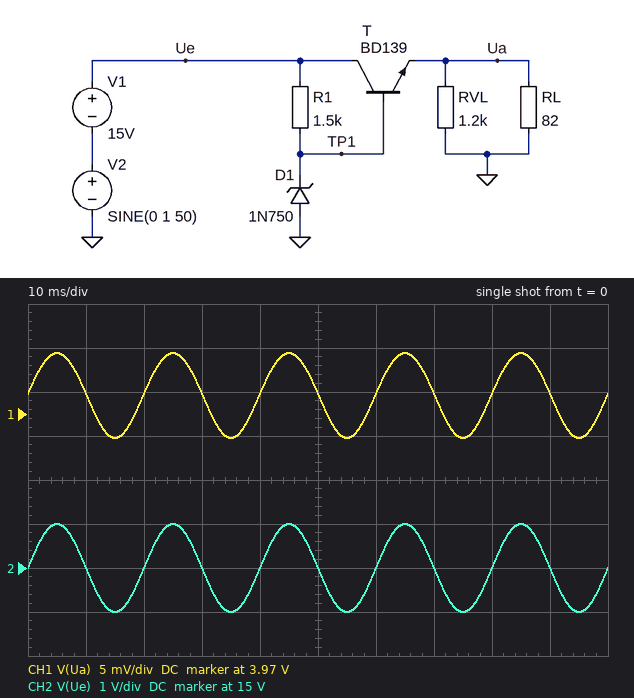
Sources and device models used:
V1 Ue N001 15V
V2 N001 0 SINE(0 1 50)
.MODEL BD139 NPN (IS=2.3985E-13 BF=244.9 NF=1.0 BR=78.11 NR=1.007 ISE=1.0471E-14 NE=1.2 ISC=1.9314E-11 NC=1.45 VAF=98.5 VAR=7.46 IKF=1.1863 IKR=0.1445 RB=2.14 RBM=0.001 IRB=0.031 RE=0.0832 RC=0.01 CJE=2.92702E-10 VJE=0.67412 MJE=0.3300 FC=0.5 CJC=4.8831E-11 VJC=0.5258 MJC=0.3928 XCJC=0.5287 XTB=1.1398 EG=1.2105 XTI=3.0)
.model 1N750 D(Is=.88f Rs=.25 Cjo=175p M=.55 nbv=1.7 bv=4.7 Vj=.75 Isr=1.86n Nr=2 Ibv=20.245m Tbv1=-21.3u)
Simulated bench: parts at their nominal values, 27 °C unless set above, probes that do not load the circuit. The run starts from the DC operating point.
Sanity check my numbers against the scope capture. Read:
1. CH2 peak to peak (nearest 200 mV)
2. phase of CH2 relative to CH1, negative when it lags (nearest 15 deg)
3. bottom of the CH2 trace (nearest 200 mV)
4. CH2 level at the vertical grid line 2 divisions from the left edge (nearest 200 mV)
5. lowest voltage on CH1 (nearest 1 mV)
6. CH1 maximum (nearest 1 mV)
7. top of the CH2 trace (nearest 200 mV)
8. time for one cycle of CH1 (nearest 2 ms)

2.0 V
0 deg
14.0 V
15.0 V
3.967 V
3.977 V
16.0 V
20 ms
